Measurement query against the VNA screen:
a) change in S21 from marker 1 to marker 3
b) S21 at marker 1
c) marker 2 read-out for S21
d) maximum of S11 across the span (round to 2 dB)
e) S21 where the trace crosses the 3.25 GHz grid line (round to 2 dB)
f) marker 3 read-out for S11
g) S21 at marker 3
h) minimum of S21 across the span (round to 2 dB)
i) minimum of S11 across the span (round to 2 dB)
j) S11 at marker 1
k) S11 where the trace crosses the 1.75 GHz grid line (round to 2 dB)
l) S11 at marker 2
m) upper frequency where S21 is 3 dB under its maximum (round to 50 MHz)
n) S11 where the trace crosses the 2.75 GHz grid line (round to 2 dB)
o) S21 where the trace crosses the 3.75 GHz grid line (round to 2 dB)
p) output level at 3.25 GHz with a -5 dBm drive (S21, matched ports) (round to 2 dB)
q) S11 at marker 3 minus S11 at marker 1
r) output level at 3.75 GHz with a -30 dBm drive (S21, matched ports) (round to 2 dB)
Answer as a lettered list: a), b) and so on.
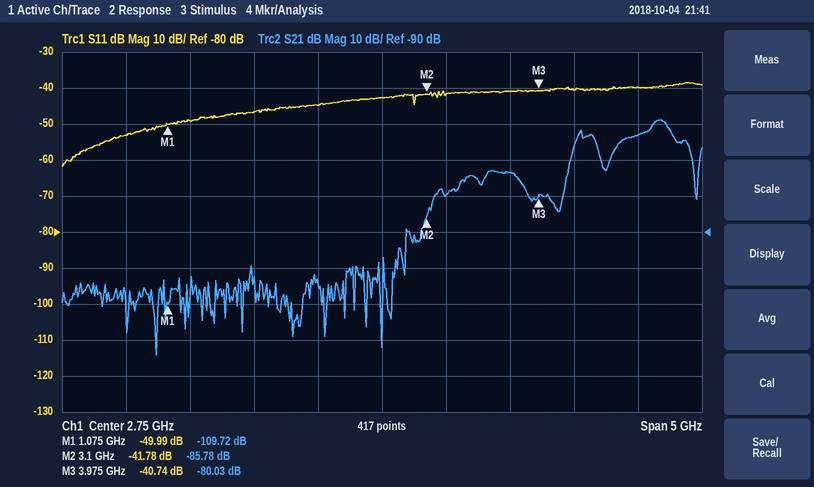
a) 29.69 dB
b) -109.72 dB
c) -85.78 dB
d) -38 dB
e) -80 dB
f) -40.74 dB
g) -80.03 dB
h) -124 dB
i) -62 dB
j) -49.99 dB
k) -46 dB
l) -41.78 dB
m) 5.00 GHz
n) -42 dB
o) -74 dB
p) -84 dBm
q) 9.25 dB
r) -104 dBm
